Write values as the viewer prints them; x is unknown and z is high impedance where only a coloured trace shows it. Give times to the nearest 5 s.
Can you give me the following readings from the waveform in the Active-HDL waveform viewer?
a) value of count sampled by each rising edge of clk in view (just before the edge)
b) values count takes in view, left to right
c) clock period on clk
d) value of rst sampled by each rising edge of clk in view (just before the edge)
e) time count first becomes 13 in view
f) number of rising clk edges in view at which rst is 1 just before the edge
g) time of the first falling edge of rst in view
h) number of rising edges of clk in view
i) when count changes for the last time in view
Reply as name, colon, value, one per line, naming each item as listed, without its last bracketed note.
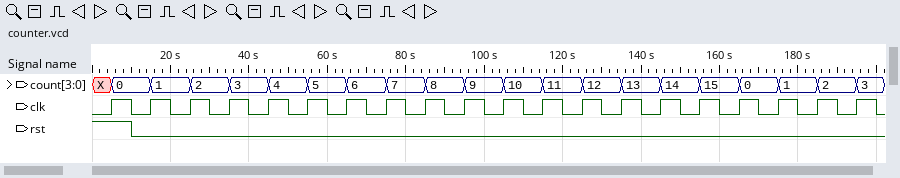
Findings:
value of count sampled by each rising edge of clk in view: X, 0, 1, 2, 3, 4, 5, 6, 7, 8, 9, 10, 11, 12, 13, 14, 15, 0, 1, 2
values count takes in view, left to right: X, 0, 1, 2, 3, 4, 5, 6, 7, 8, 9, 10, 11, 12, 13, 14, 15, 0, 1, 2, 3
clock period on clk: 10 s
value of rst sampled by each rising edge of clk in view: 1 0 0 0 0 0 0 0 0 0 0 0 0 0 0 0 0 0 0 0
time count first becomes 13 in view: 135 s
number of rising clk edges in view at which rst is 1 just before the edge: 1
time of the first falling edge of rst in view: 10 s
number of rising edges of clk in view: 20
when count changes for the last time in view: 195 s
